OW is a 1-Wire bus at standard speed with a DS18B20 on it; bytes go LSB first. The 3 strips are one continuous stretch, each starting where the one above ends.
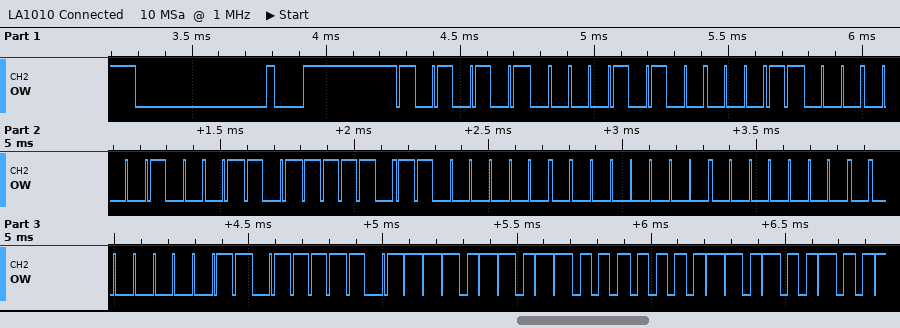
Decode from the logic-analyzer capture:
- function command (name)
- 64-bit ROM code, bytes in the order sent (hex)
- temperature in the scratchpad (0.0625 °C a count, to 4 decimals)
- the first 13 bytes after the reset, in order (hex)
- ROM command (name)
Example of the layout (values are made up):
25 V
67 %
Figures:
Read Scratchpad
28 18 88 7D 03 00 00 C0
27.4375 °C
55 28 18 88 7D 03 00 00 C0 BE B7 01 4B
Match ROM
